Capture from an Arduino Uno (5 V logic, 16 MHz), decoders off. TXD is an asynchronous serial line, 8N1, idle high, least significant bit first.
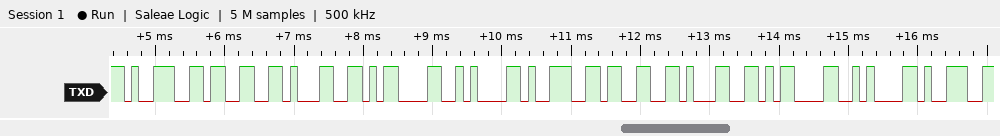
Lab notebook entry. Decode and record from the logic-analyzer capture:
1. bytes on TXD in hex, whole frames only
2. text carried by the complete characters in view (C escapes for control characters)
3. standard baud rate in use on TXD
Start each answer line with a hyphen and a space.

- 0x39 0x33 0x31 0x0D 0x0A 0x39 0x33 0x31 0x0D 0x0A 0x39
- "931\r\n931\r\n9"
- 9600 baud
